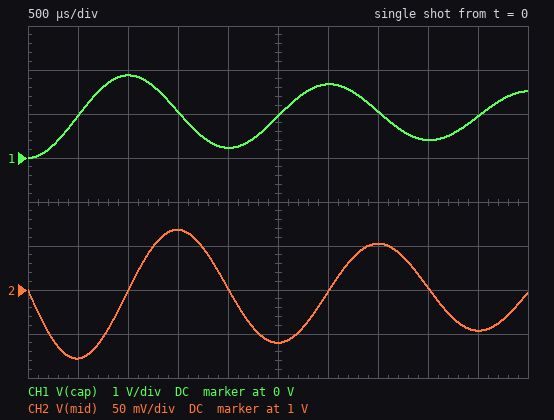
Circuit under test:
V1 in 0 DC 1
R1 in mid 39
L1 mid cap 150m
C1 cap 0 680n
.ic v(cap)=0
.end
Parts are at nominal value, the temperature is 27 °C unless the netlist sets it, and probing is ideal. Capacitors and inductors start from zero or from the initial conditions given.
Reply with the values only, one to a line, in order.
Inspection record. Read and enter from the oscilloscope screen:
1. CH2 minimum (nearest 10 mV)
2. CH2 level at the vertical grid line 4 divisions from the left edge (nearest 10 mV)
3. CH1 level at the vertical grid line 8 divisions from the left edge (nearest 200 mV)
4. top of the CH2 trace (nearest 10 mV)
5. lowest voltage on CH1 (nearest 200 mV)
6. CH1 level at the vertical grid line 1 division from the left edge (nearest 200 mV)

920 mV
1.00 V
400 mV
1.07 V
0 V
1.0 V
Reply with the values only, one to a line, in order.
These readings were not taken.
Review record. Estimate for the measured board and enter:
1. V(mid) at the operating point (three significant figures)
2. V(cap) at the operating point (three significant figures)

1.00 V
1.00 V
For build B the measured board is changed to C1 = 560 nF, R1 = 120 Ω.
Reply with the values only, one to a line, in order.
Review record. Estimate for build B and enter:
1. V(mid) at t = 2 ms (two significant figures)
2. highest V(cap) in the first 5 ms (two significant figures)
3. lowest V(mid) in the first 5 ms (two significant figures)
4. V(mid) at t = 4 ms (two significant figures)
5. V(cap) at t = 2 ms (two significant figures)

940 mV
1.7 V
800 mV
960 mV
590 mV
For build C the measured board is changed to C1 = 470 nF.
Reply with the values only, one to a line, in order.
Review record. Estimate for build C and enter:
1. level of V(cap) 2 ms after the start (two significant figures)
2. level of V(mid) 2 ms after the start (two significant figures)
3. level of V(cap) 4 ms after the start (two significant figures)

730 mV
950 mV
1.5 V
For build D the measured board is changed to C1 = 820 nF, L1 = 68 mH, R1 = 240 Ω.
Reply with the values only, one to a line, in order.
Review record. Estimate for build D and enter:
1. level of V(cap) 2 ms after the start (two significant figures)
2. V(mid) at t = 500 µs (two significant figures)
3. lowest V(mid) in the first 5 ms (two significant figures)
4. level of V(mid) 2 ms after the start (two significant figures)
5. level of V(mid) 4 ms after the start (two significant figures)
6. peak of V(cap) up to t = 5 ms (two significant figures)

980 mV
640 mV
510 mV
970 mV
1.0 V
1.2 V
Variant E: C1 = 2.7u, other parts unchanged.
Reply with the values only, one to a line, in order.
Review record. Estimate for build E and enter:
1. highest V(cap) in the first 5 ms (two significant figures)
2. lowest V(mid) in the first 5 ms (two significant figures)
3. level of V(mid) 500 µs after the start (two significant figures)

1.8 V
850 mV
890 mV
